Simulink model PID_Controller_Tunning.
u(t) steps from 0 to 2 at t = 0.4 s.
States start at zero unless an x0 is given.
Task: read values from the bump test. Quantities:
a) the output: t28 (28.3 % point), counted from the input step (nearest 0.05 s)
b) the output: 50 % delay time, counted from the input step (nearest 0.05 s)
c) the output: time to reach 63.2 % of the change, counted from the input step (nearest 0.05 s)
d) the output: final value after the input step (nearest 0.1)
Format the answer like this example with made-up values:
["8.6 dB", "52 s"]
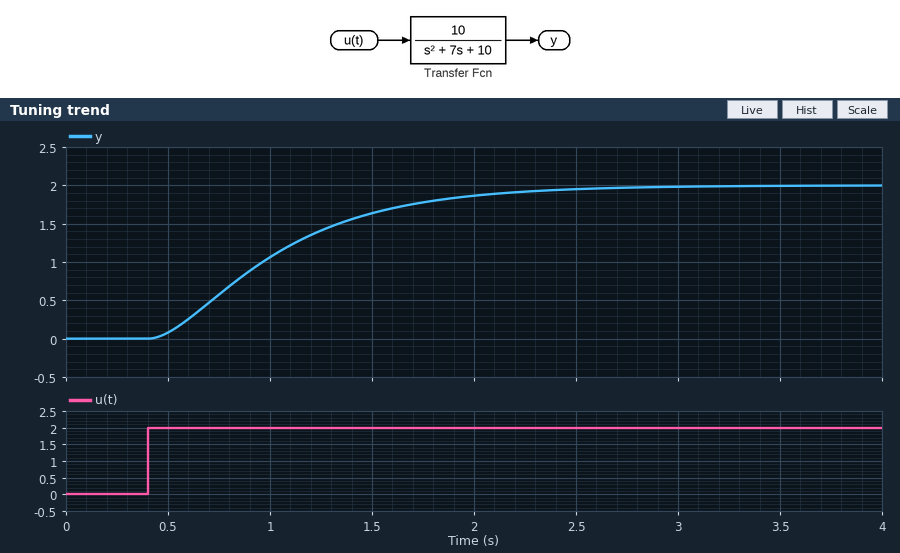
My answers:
["0.35 s", "0.55 s", "0.75 s", "2.0"]
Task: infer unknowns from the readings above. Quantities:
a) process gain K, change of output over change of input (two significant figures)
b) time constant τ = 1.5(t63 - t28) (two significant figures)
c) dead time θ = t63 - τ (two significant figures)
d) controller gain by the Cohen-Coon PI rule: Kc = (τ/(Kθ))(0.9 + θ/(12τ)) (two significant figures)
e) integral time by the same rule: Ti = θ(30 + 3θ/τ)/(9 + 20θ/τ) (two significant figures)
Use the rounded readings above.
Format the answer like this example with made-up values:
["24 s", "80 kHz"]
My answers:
["1.0", "0.60 s", "0.15 s", "3.7", "0.33 s"]
